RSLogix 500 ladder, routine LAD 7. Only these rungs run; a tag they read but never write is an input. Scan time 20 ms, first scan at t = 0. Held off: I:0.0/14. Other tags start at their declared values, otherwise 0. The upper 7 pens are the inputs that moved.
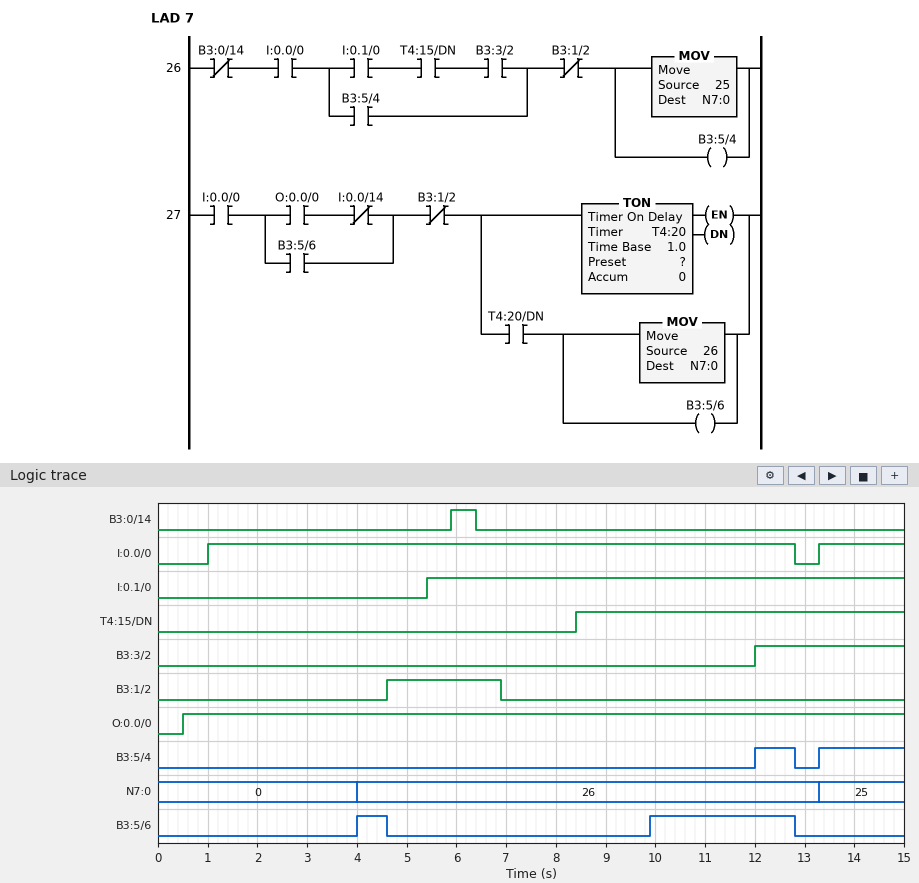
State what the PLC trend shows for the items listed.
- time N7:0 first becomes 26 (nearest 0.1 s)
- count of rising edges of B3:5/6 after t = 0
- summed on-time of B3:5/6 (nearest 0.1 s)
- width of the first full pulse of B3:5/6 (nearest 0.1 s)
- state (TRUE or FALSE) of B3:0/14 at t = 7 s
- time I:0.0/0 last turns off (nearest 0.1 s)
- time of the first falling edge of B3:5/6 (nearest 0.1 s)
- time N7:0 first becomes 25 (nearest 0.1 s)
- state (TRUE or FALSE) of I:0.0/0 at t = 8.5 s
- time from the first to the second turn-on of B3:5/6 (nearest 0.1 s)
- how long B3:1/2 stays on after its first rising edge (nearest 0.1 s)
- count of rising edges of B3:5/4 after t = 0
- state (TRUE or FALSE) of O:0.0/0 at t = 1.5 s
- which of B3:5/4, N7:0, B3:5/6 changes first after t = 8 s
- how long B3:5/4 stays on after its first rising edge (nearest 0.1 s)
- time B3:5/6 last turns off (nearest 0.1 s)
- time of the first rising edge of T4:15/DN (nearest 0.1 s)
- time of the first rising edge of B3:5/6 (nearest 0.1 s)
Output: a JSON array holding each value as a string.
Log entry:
["4.0 s", "2", "3.5 s", "0.6 s", "FALSE", "12.8 s", "4.6 s", "13.3 s", "TRUE", "5.9 s", "2.3 s", "2", "TRUE", "B3:5/6", "0.8 s", "12.8 s", "8.4 s", "4.0 s"]
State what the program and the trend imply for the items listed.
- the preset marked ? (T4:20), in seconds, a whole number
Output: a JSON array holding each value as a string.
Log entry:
["3 s"]
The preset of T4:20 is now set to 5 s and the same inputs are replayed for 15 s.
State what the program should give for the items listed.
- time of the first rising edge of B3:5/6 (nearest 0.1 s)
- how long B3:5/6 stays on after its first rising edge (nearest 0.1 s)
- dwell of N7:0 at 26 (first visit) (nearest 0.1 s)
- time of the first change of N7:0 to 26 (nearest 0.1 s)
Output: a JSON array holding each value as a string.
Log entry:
["11.9 s", "0.9 s", "1.4 s", "11.9 s"]
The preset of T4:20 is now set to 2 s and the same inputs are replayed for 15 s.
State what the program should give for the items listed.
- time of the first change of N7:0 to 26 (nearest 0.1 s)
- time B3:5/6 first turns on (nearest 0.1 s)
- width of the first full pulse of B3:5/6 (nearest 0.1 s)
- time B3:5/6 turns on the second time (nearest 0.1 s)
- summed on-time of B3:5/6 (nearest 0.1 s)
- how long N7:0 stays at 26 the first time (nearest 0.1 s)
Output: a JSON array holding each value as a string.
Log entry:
["3.0 s", "3.0 s", "1.6 s", "8.9 s", "5.5 s", "10.3 s"]
